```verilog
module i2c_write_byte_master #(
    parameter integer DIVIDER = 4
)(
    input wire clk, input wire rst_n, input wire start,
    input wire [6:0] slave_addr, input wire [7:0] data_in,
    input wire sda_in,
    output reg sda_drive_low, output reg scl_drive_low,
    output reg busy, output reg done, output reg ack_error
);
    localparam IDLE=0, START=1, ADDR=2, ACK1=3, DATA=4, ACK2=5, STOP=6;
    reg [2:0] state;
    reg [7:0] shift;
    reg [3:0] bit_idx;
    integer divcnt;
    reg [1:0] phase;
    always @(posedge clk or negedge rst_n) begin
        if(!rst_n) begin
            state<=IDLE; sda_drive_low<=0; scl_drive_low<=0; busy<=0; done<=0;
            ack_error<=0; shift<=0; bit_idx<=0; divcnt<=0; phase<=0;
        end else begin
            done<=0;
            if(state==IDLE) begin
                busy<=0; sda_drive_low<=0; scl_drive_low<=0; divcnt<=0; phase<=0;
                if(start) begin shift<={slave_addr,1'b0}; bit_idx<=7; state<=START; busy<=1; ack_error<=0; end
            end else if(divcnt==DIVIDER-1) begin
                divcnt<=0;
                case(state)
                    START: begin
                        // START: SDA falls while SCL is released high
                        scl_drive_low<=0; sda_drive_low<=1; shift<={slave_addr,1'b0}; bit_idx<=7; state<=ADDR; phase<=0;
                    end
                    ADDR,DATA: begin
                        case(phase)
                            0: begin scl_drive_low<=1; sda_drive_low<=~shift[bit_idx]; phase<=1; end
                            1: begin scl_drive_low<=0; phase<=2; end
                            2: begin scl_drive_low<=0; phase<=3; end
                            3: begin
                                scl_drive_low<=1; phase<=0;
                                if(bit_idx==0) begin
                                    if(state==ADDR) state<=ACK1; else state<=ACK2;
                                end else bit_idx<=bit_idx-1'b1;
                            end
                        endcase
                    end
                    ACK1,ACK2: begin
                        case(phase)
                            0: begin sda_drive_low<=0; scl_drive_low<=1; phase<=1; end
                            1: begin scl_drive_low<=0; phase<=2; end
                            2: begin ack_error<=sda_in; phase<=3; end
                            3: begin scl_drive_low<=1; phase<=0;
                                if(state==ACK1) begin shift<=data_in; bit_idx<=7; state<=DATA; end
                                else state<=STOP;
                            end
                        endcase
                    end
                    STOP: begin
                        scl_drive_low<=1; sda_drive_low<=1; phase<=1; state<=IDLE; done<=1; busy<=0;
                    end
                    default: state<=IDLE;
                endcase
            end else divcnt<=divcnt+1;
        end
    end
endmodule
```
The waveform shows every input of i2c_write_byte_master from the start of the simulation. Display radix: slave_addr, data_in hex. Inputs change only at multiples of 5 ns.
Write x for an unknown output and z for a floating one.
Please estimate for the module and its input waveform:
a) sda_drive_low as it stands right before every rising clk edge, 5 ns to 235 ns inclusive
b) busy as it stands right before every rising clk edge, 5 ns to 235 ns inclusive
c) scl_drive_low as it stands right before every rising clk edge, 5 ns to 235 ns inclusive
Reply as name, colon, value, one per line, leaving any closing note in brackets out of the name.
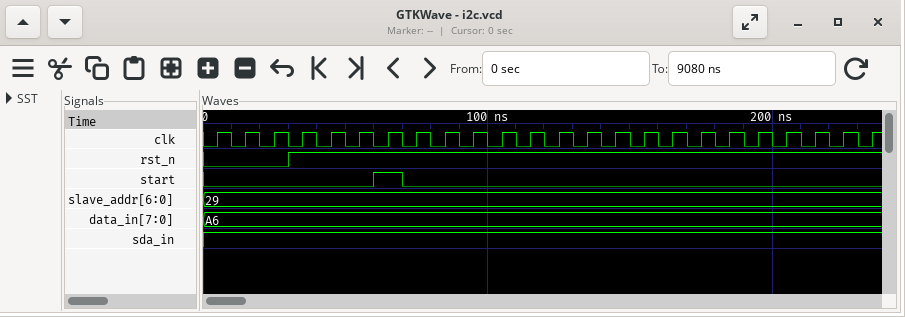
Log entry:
sda_drive_low as it stands right before every rising clk edge, 5 ns to 235 ns inclusive: 0 0 0 0 0 0 0 0 0 0 0 1 1 1 1 1 1 1 1 1 1 1 1 1
busy as it stands right before every rising clk edge, 5 ns to 235 ns inclusive: 0 0 0 0 0 0 0 1 1 1 1 1 1 1 1 1 1 1 1 1 1 1 1 1
scl_drive_low as it stands right before every rising clk edge, 5 ns to 235 ns inclusive: 0 0 0 0 0 0 0 0 0 0 0 0 0 0 0 1 1 1 1 0 0 0 0 0
